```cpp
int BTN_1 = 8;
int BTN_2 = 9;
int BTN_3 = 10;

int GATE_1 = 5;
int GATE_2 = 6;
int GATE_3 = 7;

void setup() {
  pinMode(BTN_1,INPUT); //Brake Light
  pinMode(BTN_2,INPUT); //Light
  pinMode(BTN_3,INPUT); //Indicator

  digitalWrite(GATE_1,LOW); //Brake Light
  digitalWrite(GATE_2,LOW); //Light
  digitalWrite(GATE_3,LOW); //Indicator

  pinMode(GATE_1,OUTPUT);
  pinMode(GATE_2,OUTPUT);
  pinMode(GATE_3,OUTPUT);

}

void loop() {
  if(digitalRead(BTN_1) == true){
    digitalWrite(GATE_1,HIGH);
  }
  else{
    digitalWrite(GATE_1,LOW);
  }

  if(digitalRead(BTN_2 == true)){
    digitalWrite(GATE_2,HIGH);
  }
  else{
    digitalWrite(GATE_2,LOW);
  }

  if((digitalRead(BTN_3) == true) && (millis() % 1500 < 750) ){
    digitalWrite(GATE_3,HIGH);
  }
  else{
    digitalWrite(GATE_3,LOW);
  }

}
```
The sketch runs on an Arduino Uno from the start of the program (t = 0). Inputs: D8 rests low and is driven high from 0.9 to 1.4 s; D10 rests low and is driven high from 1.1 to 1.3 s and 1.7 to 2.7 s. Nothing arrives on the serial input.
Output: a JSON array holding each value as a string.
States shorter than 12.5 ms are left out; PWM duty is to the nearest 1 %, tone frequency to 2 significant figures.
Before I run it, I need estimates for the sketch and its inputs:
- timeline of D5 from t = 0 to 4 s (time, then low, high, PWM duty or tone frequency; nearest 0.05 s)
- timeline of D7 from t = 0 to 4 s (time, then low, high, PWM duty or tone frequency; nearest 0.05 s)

["0 s low; 0.9 s high; 1.4 s low", "0 s low; 1.7 s high; 2.25 s low"]
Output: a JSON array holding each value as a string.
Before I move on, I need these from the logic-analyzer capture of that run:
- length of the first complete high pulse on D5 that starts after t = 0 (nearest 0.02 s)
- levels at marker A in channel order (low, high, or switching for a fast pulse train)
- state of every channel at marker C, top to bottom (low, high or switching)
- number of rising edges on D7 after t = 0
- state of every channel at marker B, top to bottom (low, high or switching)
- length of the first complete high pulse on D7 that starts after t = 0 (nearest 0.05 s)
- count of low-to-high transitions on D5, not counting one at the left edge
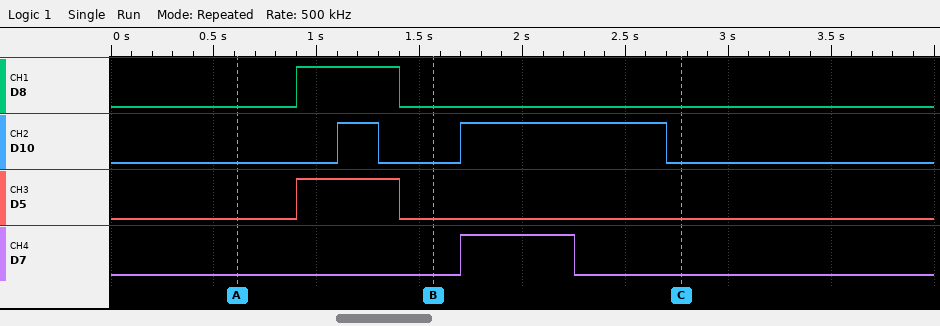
["0.50 s", "D8 low, D10 low, D5 low, D7 low", "D8 low, D10 low, D5 low, D7 low", "1", "D8 low, D10 low, D5 low, D7 low", "0.55 s", "1"]
